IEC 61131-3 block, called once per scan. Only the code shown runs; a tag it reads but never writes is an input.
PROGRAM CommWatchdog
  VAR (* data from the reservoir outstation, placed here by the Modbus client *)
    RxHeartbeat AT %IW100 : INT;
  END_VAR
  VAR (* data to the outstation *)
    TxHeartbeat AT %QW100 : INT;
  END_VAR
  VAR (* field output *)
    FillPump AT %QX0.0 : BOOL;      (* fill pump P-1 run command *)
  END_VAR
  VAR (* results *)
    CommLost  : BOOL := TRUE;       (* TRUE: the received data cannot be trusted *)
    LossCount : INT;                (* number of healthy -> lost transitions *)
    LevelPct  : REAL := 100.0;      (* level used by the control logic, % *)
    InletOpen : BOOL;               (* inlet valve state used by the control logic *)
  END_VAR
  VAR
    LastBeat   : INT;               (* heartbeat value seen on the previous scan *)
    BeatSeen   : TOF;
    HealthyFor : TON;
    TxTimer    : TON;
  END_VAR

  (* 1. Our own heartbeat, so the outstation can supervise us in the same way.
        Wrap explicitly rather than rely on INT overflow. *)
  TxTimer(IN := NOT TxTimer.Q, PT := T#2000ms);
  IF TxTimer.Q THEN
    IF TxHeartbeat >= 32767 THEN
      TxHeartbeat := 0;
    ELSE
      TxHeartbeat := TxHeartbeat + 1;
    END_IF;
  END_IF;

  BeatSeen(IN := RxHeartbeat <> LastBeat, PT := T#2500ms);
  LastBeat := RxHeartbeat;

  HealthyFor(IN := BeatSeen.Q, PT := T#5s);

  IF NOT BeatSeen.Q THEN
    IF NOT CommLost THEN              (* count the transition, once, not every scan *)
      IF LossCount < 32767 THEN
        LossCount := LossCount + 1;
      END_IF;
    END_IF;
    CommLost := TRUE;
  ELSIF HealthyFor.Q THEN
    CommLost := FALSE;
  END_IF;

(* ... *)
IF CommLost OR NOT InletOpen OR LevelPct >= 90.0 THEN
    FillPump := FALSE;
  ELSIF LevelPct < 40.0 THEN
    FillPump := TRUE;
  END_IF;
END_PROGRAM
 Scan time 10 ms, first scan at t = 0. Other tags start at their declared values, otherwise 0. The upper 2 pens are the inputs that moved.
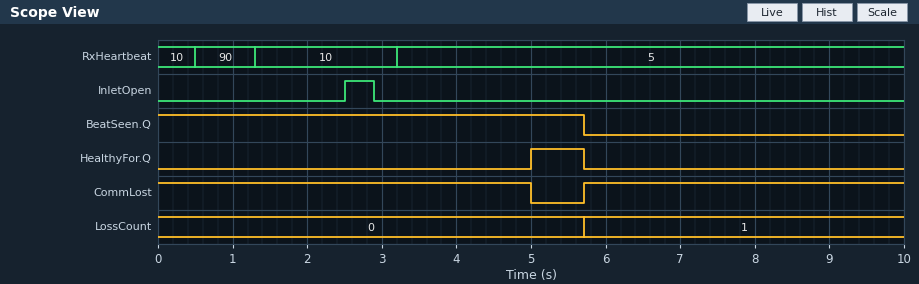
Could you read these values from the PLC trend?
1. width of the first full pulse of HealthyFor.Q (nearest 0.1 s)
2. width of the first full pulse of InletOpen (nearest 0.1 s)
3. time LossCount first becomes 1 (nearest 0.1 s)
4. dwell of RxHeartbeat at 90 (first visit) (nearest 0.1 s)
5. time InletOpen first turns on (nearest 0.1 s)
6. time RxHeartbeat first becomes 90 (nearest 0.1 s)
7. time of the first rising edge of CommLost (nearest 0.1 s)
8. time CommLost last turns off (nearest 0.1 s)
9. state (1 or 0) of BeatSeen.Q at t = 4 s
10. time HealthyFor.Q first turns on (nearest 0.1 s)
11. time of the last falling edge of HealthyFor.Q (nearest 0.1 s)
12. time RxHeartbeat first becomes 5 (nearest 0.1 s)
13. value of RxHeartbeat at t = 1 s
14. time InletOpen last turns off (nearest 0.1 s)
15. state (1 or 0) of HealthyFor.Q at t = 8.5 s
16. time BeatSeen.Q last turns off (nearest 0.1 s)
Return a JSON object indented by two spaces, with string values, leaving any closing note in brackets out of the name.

{
  "width of the first full pulse of HealthyFor.Q": "0.7 s",
  "width of the first full pulse of InletOpen": "0.4 s",
  "time LossCount first becomes 1": "5.7 s",
  "dwell of RxHeartbeat at 90 (first visit)": "0.8 s",
  "time InletOpen first turns on": "2.5 s",
  "time RxHeartbeat first becomes 90": "0.5 s",
  "time of the first rising edge of CommLost": "5.7 s",
  "time CommLost last turns off": "5.0 s",
  "state (1 or 0) of BeatSeen.Q at t = 4 s": "1",
  "time HealthyFor.Q first turns on": "5.0 s",
  "time of the last falling edge of HealthyFor.Q": "5.7 s",
  "time RxHeartbeat first becomes 5": "3.2 s",
  "value of RxHeartbeat at t = 1 s": "90",
  "time InletOpen last turns off": "2.9 s",
  "state (1 or 0) of HealthyFor.Q at t = 8.5 s": "0",
  "time BeatSeen.Q last turns off": "5.7 s"
}
